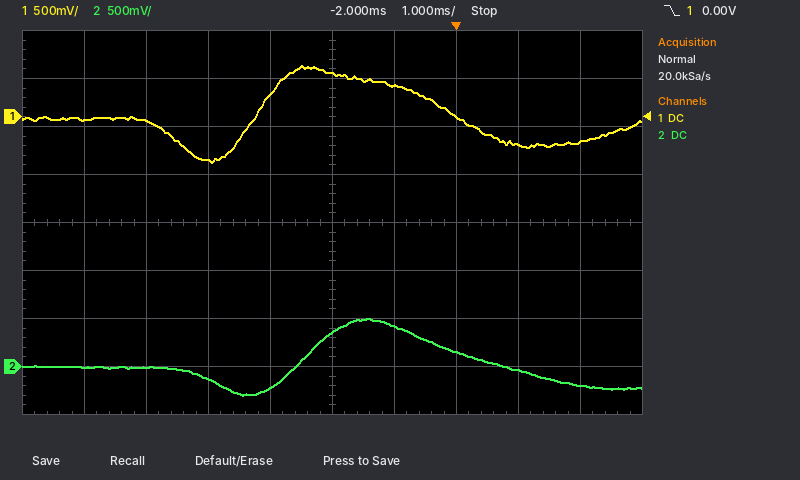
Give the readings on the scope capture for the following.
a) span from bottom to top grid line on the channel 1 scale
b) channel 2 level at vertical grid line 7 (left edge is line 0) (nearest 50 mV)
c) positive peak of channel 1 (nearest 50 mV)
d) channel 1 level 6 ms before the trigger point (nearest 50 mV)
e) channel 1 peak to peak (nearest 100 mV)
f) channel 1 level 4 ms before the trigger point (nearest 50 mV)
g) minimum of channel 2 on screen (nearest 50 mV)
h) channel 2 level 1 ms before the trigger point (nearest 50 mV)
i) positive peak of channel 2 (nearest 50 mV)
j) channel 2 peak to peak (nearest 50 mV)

4 V
150 mV
550 mV
-50 mV
1.00 V
-450 mV
-300 mV
400 mV
500 mV
800 mV
